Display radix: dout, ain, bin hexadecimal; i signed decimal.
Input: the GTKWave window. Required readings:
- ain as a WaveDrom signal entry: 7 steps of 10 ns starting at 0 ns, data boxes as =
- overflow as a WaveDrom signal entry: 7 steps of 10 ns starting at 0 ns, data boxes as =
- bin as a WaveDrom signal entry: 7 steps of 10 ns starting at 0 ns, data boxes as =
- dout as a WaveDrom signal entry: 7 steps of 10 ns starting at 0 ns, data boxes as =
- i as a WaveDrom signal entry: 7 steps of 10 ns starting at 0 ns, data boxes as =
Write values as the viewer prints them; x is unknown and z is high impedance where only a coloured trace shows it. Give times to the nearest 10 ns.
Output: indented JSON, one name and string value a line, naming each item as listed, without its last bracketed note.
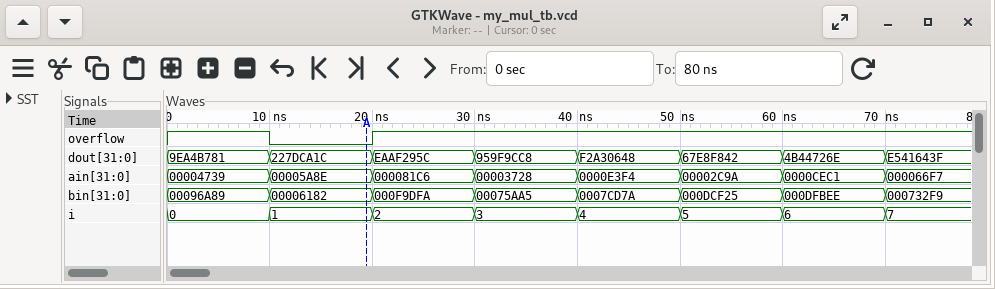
{
  "ain as a WaveDrom signal entry: 7 steps of 10 ns starting at 0 ns, data boxes as =": "{name: 'ain', wave: '=======', data: '00004739 00005A8E 000081C6 00003728 0000E3F4 00002C9A 0000CEC1'}",
  "overflow as a WaveDrom signal entry: 7 steps of 10 ns starting at 0 ns, data boxes as =": "{name: 'overflow', wave: '101....'}",
  "bin as a WaveDrom signal entry: 7 steps of 10 ns starting at 0 ns, data boxes as =": "{name: 'bin', wave: '=======', data: '00096A89 00006182 000F9DFA 00075AA5 0007CD7A 000DCF25 000DFBEE'}",
  "dout as a WaveDrom signal entry: 7 steps of 10 ns starting at 0 ns, data boxes as =": "{name: 'dout', wave: '=======', data: '9EA4B781 227DCA1C EAAF295C 959F9CC8 F2A30648 67E8F842 4B44726E'}",
  "i as a WaveDrom signal entry: 7 steps of 10 ns starting at 0 ns, data boxes as =": "{name: 'i', wave: '=======', data: '0 1 2 3 4 5 6'}"
}
